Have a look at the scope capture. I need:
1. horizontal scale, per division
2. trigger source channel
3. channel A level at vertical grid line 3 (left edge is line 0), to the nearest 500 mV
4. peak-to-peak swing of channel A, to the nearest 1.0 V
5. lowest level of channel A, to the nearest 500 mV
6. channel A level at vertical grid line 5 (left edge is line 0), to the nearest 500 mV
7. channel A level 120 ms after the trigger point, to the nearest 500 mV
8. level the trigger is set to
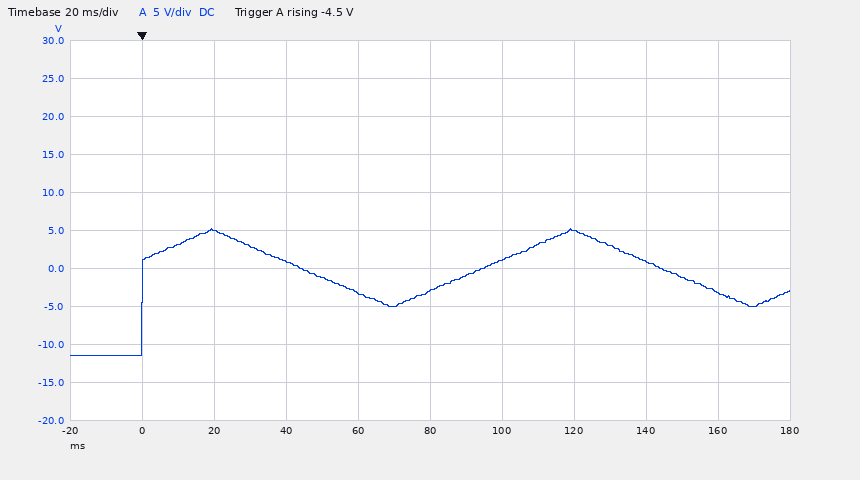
20 ms
channel A
1.0 V
17.0 V
-11.5 V
-3.0 V
5.0 V
-4.5 V
